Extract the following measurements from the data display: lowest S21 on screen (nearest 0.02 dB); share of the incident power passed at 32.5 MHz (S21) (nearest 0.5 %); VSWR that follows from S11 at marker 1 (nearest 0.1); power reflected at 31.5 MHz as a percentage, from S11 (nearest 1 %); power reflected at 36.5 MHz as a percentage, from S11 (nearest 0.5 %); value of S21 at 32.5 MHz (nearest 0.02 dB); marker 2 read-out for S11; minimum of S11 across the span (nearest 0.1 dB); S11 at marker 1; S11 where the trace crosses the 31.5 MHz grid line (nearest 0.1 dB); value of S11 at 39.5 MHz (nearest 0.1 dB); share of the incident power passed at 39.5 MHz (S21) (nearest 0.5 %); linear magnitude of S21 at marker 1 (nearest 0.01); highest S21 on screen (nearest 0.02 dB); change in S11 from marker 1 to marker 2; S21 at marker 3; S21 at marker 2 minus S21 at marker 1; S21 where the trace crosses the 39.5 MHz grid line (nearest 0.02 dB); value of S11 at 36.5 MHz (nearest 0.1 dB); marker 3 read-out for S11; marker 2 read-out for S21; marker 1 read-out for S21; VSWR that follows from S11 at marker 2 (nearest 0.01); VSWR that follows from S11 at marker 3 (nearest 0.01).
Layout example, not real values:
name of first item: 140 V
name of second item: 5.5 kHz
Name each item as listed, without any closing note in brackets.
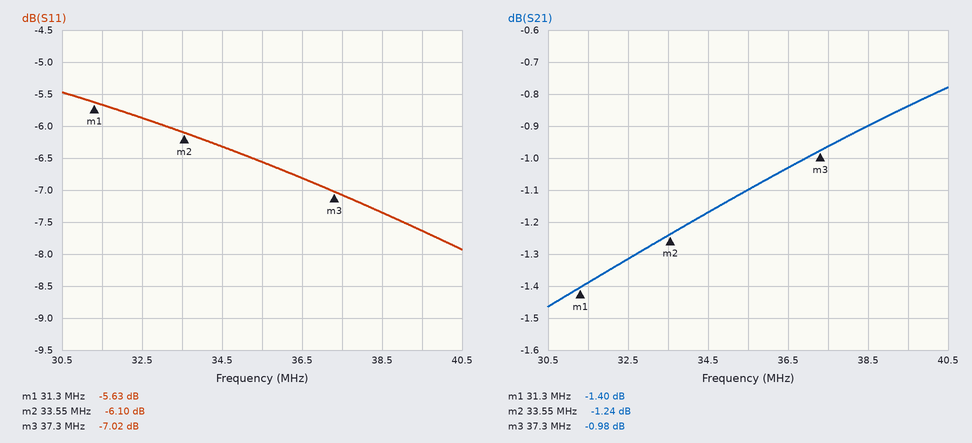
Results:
lowest S21 on screen: -1.46 dB
share of the incident power passed at 32.5 MHz (S21): 74.0 %
VSWR that follows from S11 at marker 1: 3.2
power reflected at 31.5 MHz as a percentage, from S11: 27 %
power reflected at 36.5 MHz as a percentage, from S11: 21.0 %
value of S21 at 32.5 MHz: -1.32 dB
marker 2 read-out for S11: -6.10 dB
minimum of S11 across the span: -7.9 dB
S11 at marker 1: -5.63 dB
S11 where the trace crosses the 31.5 MHz grid line: -5.7 dB
value of S11 at 39.5 MHz: -7.6 dB
share of the incident power passed at 39.5 MHz (S21): 82.5 %
linear magnitude of S21 at marker 1: 0.85
highest S21 on screen: -0.78 dB
change in S11 from marker 1 to marker 2: -0.47 dB
S21 at marker 3: -0.98 dB
S21 at marker 2 minus S21 at marker 1: 0.16 dB
S21 where the trace crosses the 39.5 MHz grid line: -0.84 dB
value of S11 at 36.5 MHz: -6.8 dB
marker 3 read-out for S11: -7.02 dB
marker 2 read-out for S21: -1.24 dB
marker 1 read-out for S21: -1.40 dB
VSWR that follows from S11 at marker 2: 2.96
VSWR that follows from S11 at marker 3: 2.61
